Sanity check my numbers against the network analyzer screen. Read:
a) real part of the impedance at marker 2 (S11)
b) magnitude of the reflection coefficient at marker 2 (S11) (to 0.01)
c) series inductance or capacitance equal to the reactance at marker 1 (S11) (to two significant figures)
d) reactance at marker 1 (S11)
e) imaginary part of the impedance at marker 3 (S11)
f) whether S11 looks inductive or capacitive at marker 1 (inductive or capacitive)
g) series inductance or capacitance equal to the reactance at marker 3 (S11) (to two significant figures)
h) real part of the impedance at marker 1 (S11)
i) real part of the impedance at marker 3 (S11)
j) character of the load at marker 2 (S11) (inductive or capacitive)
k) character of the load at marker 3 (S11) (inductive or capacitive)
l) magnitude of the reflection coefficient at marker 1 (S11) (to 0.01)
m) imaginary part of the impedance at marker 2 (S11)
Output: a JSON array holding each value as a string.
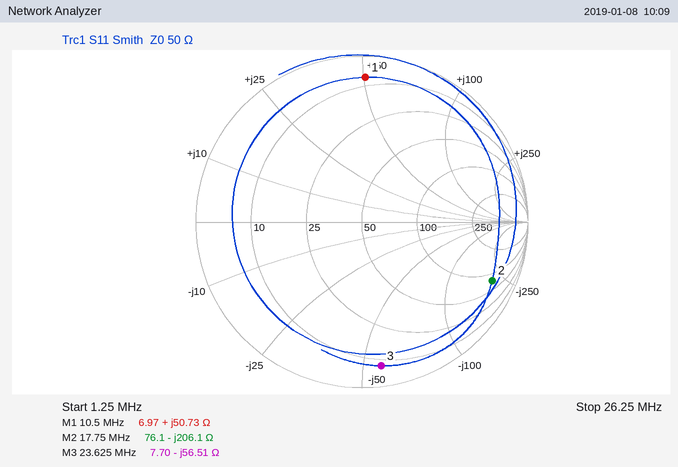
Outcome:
["76.1 Ω", "0.86", "770 nH", "+50.73 Ω", "-56.51 Ω", "inductive", "120 pF", "6.97 Ω", "7.70 Ω", "capacitive", "capacitive", "0.87", "-206.1 Ω"]
